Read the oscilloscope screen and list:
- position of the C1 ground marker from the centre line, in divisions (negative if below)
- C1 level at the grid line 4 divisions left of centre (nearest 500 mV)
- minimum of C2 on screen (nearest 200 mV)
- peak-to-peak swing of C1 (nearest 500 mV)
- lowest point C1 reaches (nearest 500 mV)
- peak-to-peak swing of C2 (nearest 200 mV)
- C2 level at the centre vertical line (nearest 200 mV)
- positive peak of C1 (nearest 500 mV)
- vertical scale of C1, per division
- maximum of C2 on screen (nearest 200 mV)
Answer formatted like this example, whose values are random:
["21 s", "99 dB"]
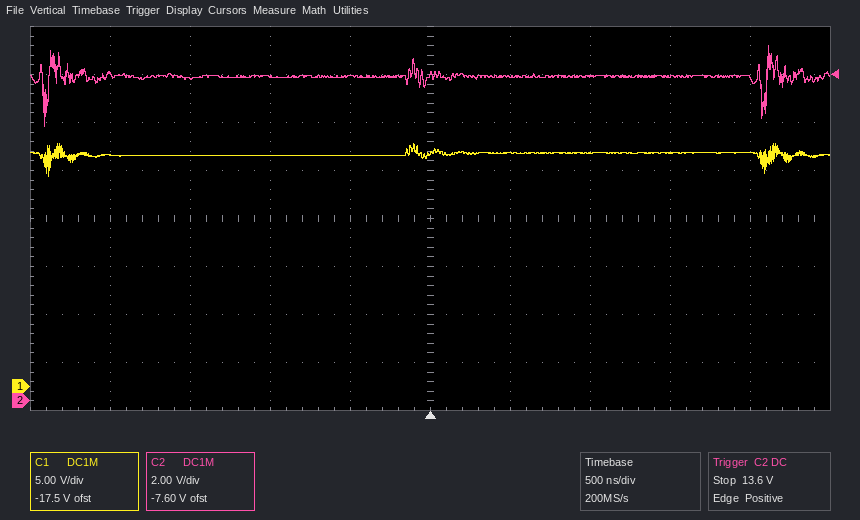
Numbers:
["-3.5 div", "24.0 V", "11.4 V", "3.5 V", "22.0 V", "3.4 V", "13.6 V", "25.5 V", "5 V", "14.8 V"]
